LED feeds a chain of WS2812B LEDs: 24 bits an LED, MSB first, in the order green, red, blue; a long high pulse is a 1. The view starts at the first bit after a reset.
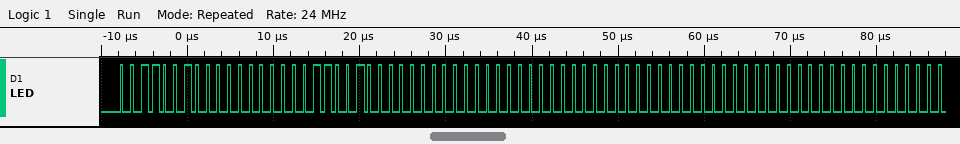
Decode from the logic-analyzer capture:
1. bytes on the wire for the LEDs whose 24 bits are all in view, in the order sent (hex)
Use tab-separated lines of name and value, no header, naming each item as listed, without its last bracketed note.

bytes on the wire for the LEDs whose 24 bits are all in view, in the order sent	32 00 32 00 00 00 00 00 00
